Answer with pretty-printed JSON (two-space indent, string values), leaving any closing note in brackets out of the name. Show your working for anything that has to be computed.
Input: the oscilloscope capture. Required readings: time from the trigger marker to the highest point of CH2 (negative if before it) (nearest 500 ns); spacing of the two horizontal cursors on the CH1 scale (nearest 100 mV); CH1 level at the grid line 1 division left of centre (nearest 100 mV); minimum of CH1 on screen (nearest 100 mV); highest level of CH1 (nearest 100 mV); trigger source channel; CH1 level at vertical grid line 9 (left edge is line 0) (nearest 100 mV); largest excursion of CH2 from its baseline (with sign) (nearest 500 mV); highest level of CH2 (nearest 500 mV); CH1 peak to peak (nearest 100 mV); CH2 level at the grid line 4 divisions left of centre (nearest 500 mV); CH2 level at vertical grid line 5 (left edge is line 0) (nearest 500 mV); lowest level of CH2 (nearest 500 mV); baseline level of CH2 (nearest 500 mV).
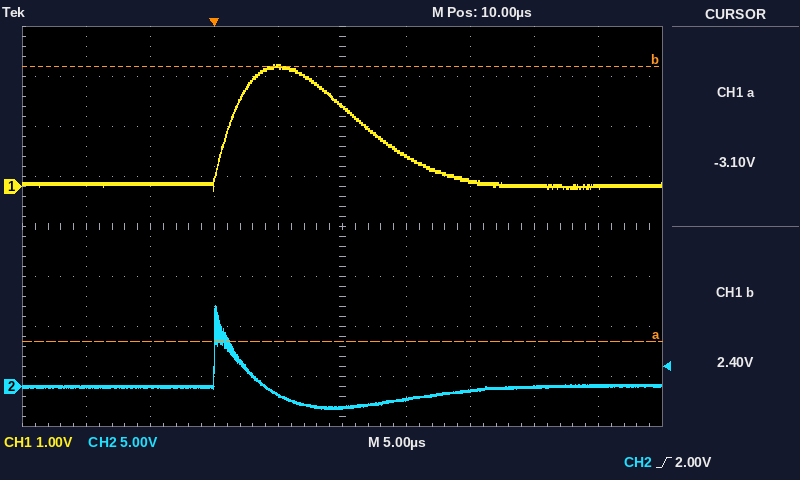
{
  "time from the trigger marker to the highest point of CH2 (negative if before it)": "0.0 µs",
  "spacing of the two horizontal cursors on the CH1 scale": "5.5 V",
  "CH1 level at the grid line 1 division left of centre": "2.4 V",
  "minimum of CH1 on screen": "-100 mV",
  "highest level of CH1": "2.4 V",
  "trigger source channel": "CH2",
  "CH1 level at vertical grid line 9 (left edge is line 0)": "0.0 V",
  "largest excursion of CH2 from its baseline (with sign)": "8.0 V − (0.0 V) = +8.0 V",
  "highest level of CH2": "8.0 V",
  "CH1 peak to peak": "2.4 V − (-100 mV) = 2.5 V",
  "CH2 level at the grid line 4 divisions left of centre": "0.0 V",
  "CH2 level at vertical grid line 5 (left edge is line 0)": "-2.0 V",
  "lowest level of CH2": "-2.0 V",
  "baseline level of CH2": "0.0 V"
}
